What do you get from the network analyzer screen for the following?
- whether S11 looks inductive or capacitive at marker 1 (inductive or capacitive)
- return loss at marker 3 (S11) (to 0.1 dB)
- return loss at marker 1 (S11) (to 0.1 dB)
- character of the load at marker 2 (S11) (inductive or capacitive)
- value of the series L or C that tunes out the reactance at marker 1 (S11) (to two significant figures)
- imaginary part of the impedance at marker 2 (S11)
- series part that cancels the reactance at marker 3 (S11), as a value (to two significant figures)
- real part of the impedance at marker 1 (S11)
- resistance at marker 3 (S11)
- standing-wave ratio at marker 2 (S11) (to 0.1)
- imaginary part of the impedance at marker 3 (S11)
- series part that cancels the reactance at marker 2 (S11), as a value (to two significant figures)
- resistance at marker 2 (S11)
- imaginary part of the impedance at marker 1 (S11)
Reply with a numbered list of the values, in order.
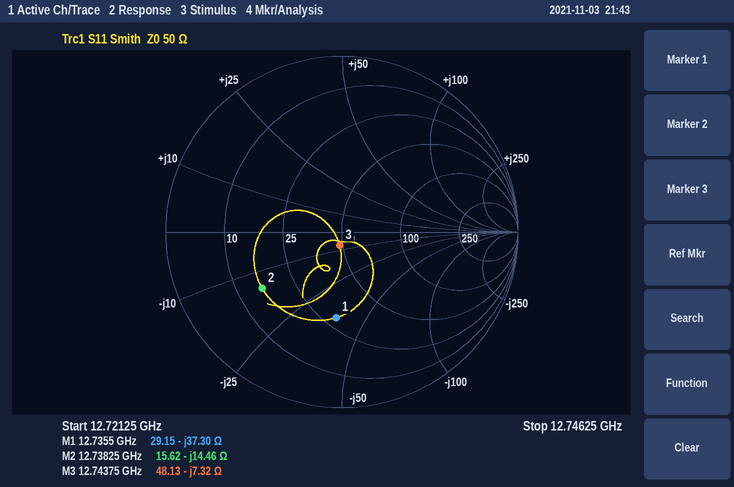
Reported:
1. capacitive
2. 22.3 dB
3. 6.2 dB
4. capacitive
5. 470 pH
6. -14.46 Ω
7. 91 pH
8. 29.15 Ω
9. 48.13 Ω
10. 3.5
11. -7.32 Ω
12. 180 pH
13. 15.62 Ω
14. -37.30 Ω
